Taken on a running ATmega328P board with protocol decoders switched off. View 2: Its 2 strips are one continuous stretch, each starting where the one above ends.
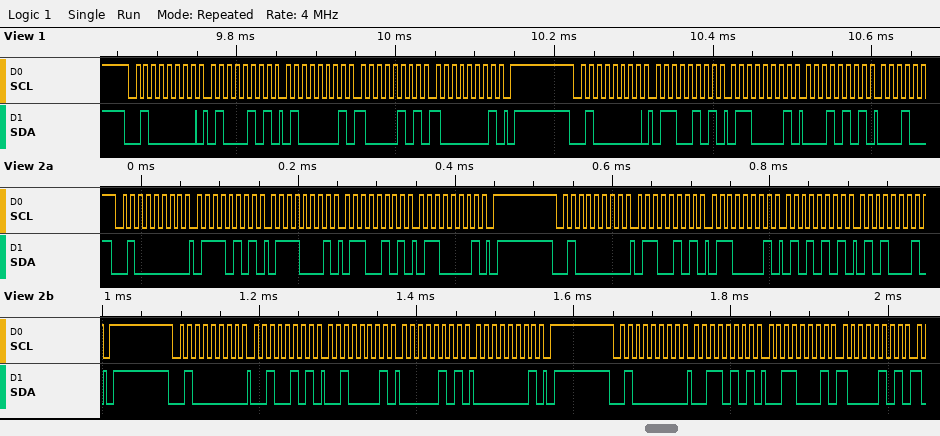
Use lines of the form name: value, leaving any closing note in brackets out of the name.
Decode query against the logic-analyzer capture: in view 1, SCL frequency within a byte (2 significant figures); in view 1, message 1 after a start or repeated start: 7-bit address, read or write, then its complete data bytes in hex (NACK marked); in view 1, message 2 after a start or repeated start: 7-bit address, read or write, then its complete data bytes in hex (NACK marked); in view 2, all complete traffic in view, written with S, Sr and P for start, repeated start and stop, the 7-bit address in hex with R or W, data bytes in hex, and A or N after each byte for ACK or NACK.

in view 1, SCL frequency within a byte: 100 kHz
in view 1, message 1 after a start or repeated start: 7-bit address, read or write, then its complete data bytes in hex: 0x20 write: 45 41 85 81
in view 1, message 2 after a start or repeated start: 7-bit address, read or write, then its complete data bytes in hex: 0x20 write: 65 61 15
in view 2, all complete traffic in view, written with S, Sr and P for start, repeated start and stop, the 7-bit address in hex with R or W, data bytes in hex, and A or N after each byte for ACK or NACK: S 20W A 75 A 71 A 65 A 61 A P S 20W A 65 A 61 A 55 A 51 A P S 20W A 25 A 21 A 05 A 01 A P S 20W A 35 A 31 A 85 A
